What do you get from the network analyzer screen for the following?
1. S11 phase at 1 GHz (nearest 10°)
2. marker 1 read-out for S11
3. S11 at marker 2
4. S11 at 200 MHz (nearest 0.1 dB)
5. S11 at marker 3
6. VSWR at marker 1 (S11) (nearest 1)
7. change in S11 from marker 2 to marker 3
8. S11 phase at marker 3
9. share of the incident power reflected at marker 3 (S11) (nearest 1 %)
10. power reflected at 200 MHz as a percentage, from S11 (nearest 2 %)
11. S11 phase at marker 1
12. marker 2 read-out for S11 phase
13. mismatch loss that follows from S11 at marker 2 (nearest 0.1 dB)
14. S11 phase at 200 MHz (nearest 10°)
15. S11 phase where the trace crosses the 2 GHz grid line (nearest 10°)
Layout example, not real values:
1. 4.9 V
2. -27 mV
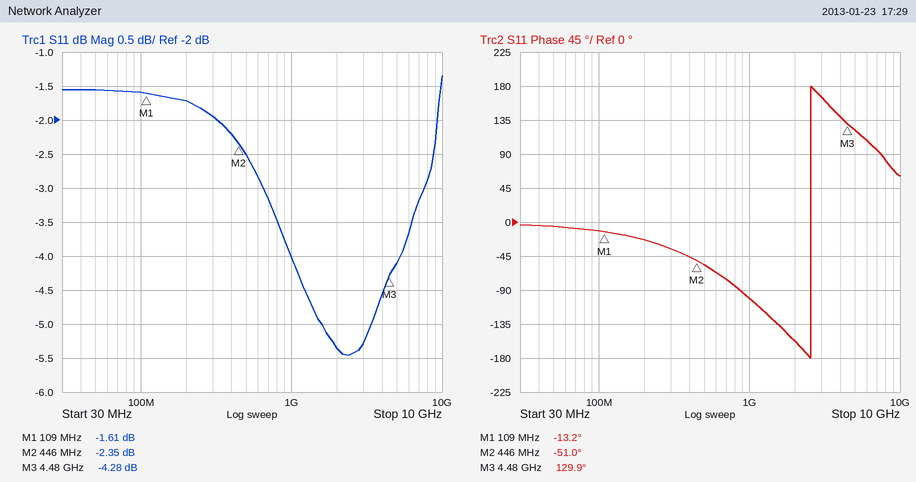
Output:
1. -100°
2. -1.61 dB
3. -2.35 dB
4. -1.7 dB
5. -4.28 dB
6. 11
7. -1.93 dB
8. 129.9°
9. 37 %
10. 68 %
11. -13.2°
12. -51.0°
13. 3.8 dB
14. -20°
15. -160°
